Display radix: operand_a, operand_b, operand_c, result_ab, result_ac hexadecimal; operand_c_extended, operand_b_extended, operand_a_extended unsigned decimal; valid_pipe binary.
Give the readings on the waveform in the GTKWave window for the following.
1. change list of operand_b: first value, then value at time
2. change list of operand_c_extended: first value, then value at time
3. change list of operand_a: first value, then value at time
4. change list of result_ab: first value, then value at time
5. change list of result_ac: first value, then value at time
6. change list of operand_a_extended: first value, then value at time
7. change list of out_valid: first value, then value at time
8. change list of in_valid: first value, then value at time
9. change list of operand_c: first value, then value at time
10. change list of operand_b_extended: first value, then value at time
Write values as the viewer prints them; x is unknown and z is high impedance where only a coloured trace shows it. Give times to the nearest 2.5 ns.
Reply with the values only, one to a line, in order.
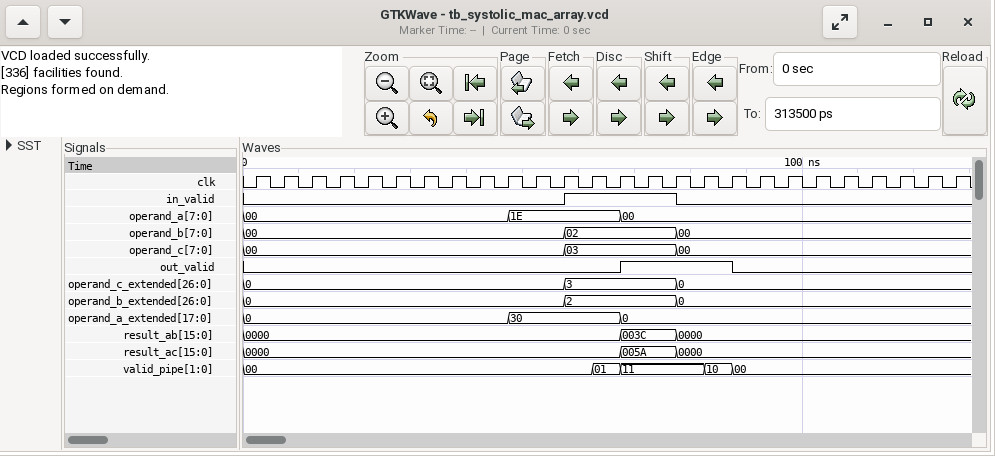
00, 02 at 57.5 ns, 00 at 77.5 ns
0, 3 at 57.5 ns, 0 at 77.5 ns
00, 1E at 47.5 ns, 00 at 67.5 ns
0000, 003C at 67.5 ns, 0000 at 77.5 ns
0000, 005A at 67.5 ns, 0000 at 77.5 ns
0, 30 at 47.5 ns, 0 at 67.5 ns
0, 1 at 67.5 ns, 0 at 87.5 ns
0, 1 at 57.5 ns, 0 at 77.5 ns
00, 03 at 57.5 ns, 00 at 77.5 ns
0, 2 at 57.5 ns, 0 at 77.5 ns
